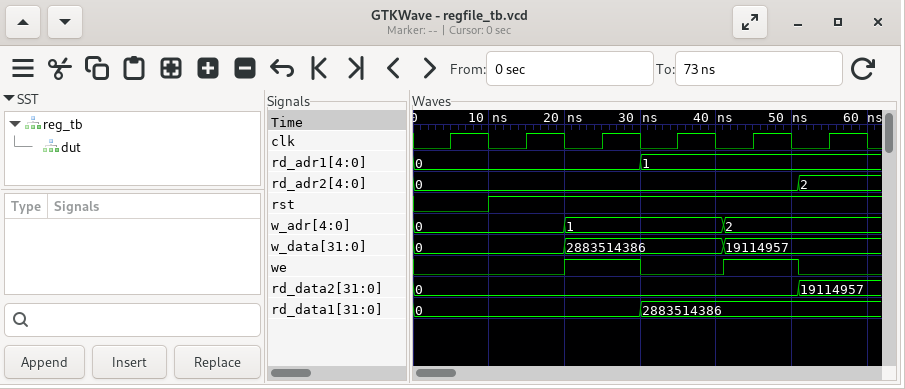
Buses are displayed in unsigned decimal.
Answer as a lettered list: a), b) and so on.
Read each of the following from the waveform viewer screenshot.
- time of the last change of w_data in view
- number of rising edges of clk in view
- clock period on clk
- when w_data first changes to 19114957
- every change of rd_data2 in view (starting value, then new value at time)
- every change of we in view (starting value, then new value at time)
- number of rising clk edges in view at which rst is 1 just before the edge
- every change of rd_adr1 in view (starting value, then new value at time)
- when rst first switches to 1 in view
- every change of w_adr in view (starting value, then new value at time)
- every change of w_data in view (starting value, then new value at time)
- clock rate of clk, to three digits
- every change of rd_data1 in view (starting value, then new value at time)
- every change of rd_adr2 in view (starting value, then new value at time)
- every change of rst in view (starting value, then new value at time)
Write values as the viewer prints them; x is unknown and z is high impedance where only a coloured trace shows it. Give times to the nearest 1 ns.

a) 41 ns
b) 6
c) 10 ns
d) 41 ns
e) 0, 19114957 at 51 ns
f) 0, 1 at 20 ns, 0 at 30 ns, 1 at 41 ns, 0 at 51 ns
g) 5
h) 0, 1 at 30 ns
i) 10 ns
j) 0, 1 at 20 ns, 2 at 41 ns
k) 0, 2883514386 at 20 ns, 19114957 at 41 ns
l) 100 MHz
m) 0, 2883514386 at 30 ns
n) 0, 2 at 51 ns
o) 0, 1 at 10 ns
